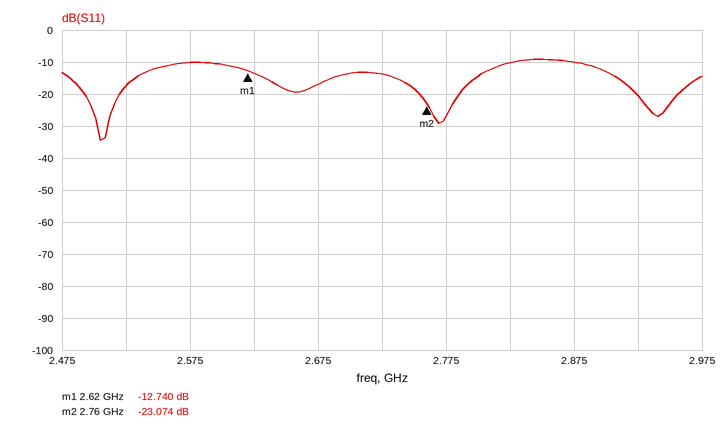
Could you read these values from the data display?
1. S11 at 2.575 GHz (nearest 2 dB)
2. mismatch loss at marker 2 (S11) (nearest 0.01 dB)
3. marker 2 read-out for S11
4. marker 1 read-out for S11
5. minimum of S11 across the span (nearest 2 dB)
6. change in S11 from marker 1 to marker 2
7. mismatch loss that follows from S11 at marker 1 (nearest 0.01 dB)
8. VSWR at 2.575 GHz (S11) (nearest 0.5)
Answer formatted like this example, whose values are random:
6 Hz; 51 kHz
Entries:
-10 dB; 0.02 dB; -23.074 dB; -12.740 dB; -34 dB; -10.334 dB; 0.24 dB; 2.0
